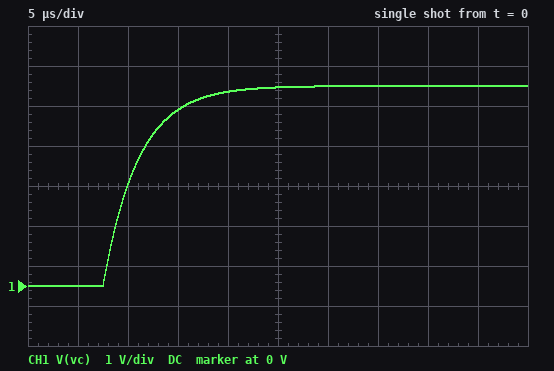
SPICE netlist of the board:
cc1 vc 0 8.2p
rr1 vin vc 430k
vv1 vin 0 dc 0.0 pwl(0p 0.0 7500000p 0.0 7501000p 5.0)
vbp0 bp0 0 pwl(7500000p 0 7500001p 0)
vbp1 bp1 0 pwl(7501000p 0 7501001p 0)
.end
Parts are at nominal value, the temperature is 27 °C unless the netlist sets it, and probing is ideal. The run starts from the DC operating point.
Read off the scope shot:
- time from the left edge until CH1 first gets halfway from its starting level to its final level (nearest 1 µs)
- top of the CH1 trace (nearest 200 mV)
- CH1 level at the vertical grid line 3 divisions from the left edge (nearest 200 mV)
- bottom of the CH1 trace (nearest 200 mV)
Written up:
10 µs
5.0 V
4.4 V
0 V
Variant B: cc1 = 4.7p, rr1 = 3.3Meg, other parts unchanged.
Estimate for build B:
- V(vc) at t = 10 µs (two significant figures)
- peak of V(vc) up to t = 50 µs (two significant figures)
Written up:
740 mV
4.7 V
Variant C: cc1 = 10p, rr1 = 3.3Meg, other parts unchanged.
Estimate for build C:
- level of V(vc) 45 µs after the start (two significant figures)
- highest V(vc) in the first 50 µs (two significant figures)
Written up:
3.4 V
3.6 V
